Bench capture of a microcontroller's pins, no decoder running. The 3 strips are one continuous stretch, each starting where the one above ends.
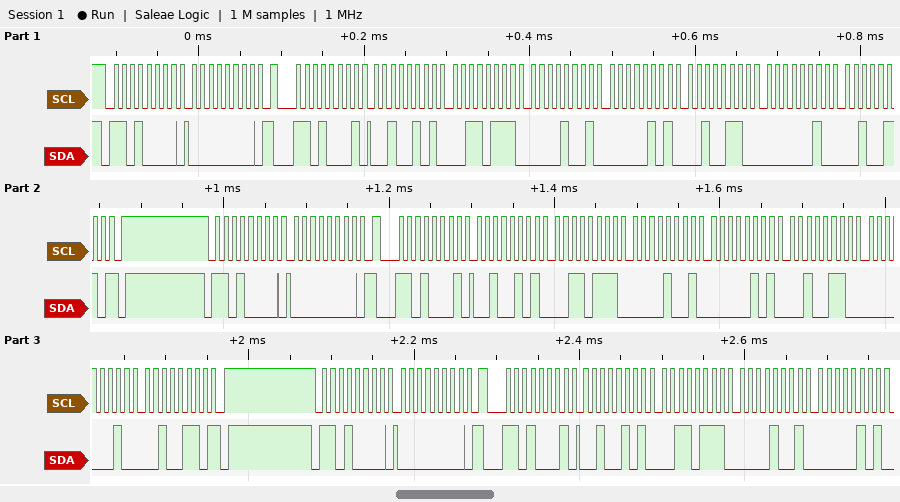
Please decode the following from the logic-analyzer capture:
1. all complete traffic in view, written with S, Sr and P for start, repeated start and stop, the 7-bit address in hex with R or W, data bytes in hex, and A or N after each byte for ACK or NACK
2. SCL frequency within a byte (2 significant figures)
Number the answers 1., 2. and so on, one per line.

1. S 68W A 00 A Sr 68R A 25 A 37 A 09 A 05 A 26 A 02 A 26 N P S 68W A 00 A Sr 68R A 25 A 37 A 09 A 05 A 26 A 02 A 26 N P S 68W A 00 A Sr 68R A 25 A 37 A 09 A 05 A
2. 100 kHz
